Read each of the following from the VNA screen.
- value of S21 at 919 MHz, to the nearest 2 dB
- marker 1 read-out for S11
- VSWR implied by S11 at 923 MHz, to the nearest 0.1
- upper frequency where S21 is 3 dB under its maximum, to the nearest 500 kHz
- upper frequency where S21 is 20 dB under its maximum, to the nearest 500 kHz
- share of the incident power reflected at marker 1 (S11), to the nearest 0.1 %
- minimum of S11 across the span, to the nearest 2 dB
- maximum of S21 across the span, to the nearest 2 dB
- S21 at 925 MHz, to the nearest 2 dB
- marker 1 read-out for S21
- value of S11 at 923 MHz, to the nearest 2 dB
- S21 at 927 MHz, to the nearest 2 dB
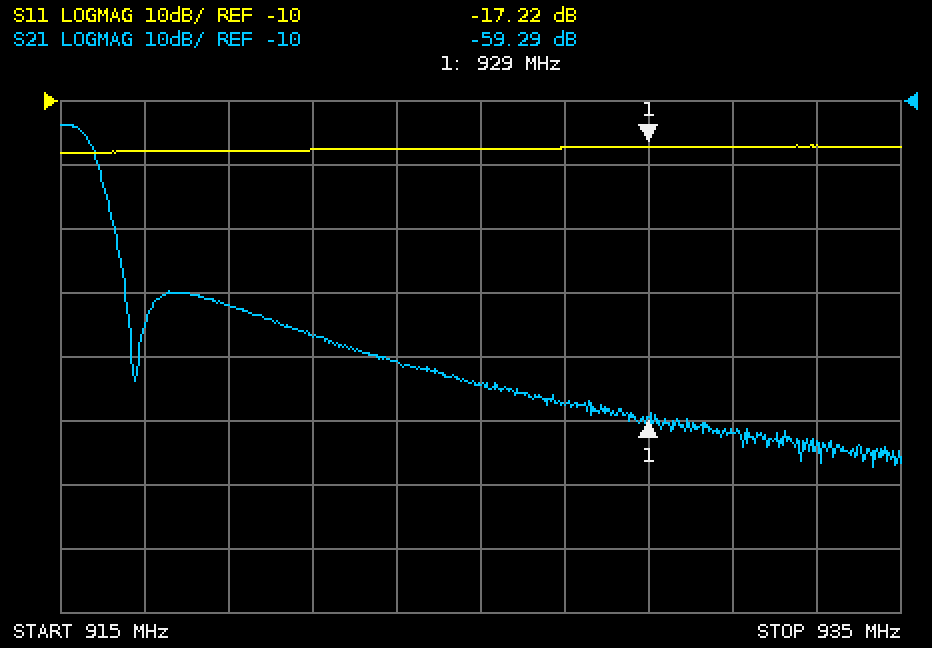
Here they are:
-42 dB
-17.22 dB
1.3
915.5 MHz
916.5 MHz
1.9 %
-18 dB
-14 dB
-54 dB
-59.29 dB
-18 dB
-58 dB
